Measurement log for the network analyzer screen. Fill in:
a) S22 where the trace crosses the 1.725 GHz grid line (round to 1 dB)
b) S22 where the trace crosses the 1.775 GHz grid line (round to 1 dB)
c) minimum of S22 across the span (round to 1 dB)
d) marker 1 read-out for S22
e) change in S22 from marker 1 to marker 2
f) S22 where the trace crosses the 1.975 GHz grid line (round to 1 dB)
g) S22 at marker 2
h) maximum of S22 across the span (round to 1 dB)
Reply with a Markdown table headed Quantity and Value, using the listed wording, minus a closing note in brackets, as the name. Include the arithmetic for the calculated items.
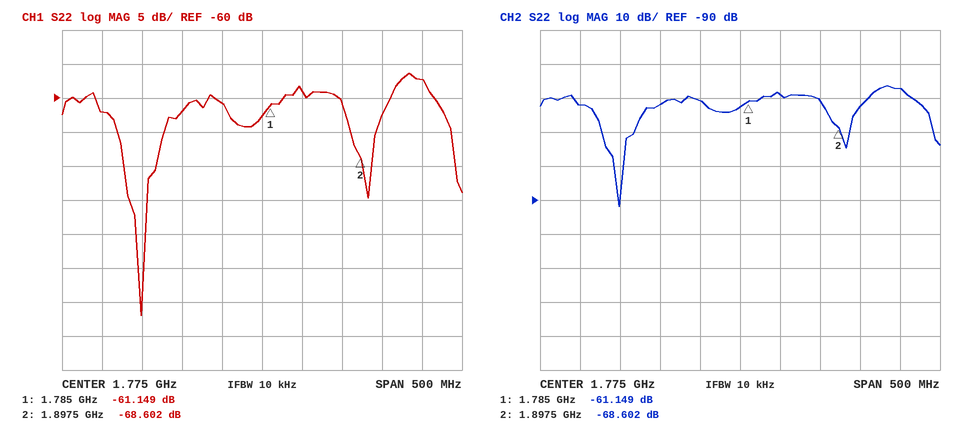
| Quantity | Value |
|---|---|
| S22 where the trace crosses the 1.725 GHz grid line | -61 dB |
| S22 where the trace crosses the 1.775 GHz grid line | -63 dB |
| minimum of S22 across the span | -92 dB |
| marker 1 read-out for S22 | -61.149 dB |
| change in S22 from marker 1 to marker 2 | -68.602 − (-61.149) = -7.453 dB |
| S22 where the trace crosses the 1.975 GHz grid line | -57 dB |
| S22 at marker 2 | -68.602 dB |
| maximum of S22 across the span | -56 dB |
